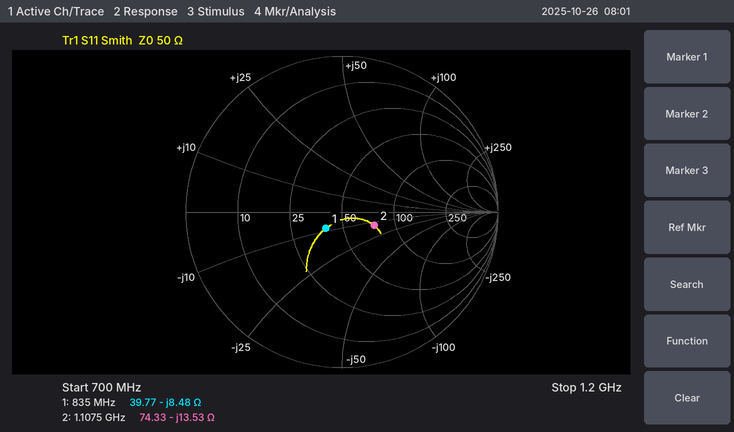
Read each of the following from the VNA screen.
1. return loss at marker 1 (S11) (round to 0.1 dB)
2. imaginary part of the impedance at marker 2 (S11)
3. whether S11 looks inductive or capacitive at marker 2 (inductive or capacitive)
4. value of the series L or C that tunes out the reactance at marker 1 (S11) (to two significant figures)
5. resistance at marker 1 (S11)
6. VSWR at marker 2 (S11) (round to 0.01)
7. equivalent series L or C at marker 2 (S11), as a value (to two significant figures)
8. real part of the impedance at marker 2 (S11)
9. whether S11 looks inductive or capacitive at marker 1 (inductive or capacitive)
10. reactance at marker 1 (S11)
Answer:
16.6 dB
-13.53 Ω
capacitive
1.6 nH
39.77 Ω
1.57
11 pF
74.33 Ω
capacitive
-8.48 Ω
